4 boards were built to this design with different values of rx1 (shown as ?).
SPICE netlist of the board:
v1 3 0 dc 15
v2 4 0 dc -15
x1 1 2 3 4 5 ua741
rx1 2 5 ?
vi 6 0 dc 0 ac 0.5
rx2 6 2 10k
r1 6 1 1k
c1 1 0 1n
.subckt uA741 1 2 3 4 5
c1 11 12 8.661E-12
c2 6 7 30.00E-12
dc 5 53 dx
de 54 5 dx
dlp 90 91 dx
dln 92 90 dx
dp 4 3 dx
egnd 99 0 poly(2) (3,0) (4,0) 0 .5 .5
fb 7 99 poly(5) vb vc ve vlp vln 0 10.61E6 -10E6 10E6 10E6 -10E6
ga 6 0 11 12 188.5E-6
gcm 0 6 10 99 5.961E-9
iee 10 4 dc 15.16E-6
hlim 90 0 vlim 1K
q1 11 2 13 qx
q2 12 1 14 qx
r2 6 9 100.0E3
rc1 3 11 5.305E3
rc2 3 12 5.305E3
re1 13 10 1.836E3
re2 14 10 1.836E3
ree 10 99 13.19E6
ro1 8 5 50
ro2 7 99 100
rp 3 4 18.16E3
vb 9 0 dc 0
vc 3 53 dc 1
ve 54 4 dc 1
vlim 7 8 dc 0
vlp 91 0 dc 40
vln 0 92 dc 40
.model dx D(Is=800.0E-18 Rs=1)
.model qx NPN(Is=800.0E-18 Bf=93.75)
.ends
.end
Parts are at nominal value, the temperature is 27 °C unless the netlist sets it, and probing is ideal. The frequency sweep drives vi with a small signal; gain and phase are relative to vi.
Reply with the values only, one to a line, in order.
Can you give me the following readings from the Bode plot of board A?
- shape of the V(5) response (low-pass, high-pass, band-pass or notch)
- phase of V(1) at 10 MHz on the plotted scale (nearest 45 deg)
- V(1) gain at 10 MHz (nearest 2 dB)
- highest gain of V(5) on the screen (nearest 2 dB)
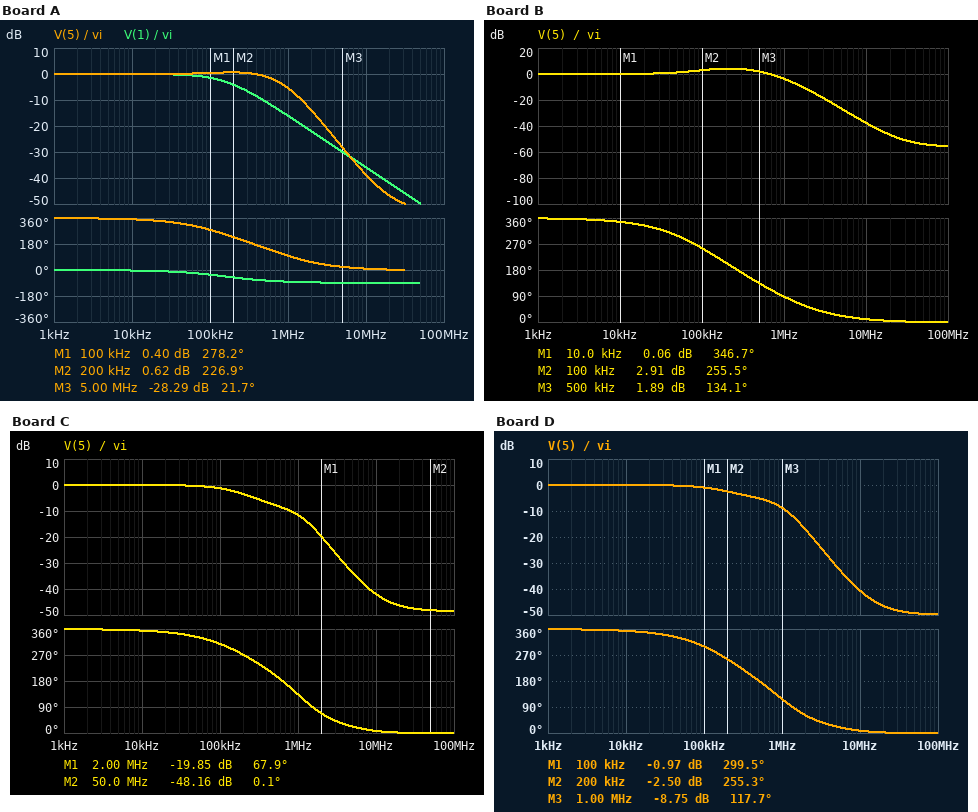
low-pass
-90 deg
-36 dB
0 dB
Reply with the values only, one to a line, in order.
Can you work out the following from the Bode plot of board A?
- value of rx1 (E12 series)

12 kΩ
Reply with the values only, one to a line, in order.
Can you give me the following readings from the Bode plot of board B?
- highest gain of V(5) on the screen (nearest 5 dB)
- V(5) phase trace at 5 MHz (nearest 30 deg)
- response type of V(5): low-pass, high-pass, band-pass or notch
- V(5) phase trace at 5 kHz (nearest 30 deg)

5 dB
30 deg
low-pass
360 deg
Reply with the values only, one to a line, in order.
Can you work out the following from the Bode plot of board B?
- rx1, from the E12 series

22 kΩ
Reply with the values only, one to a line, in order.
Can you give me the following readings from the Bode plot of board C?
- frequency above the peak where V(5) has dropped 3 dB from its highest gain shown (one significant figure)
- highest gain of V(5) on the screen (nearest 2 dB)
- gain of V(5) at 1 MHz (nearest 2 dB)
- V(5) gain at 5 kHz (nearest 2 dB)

200 kHz
0 dB
-12 dB
0 dB
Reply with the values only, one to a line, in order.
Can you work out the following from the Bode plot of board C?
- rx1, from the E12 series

3.3 kΩ
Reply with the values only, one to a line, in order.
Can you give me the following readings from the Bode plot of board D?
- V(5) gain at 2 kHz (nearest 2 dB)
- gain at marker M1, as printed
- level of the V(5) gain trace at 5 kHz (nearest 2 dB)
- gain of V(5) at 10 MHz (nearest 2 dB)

0 dB
-0.97 dB
0 dB
-40 dB
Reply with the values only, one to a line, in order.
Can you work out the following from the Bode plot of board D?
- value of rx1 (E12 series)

5.6 kΩ
